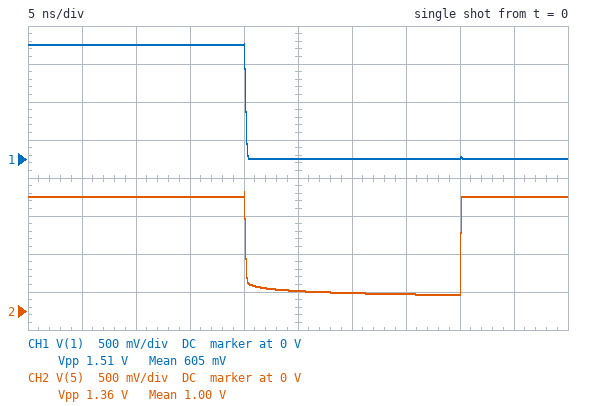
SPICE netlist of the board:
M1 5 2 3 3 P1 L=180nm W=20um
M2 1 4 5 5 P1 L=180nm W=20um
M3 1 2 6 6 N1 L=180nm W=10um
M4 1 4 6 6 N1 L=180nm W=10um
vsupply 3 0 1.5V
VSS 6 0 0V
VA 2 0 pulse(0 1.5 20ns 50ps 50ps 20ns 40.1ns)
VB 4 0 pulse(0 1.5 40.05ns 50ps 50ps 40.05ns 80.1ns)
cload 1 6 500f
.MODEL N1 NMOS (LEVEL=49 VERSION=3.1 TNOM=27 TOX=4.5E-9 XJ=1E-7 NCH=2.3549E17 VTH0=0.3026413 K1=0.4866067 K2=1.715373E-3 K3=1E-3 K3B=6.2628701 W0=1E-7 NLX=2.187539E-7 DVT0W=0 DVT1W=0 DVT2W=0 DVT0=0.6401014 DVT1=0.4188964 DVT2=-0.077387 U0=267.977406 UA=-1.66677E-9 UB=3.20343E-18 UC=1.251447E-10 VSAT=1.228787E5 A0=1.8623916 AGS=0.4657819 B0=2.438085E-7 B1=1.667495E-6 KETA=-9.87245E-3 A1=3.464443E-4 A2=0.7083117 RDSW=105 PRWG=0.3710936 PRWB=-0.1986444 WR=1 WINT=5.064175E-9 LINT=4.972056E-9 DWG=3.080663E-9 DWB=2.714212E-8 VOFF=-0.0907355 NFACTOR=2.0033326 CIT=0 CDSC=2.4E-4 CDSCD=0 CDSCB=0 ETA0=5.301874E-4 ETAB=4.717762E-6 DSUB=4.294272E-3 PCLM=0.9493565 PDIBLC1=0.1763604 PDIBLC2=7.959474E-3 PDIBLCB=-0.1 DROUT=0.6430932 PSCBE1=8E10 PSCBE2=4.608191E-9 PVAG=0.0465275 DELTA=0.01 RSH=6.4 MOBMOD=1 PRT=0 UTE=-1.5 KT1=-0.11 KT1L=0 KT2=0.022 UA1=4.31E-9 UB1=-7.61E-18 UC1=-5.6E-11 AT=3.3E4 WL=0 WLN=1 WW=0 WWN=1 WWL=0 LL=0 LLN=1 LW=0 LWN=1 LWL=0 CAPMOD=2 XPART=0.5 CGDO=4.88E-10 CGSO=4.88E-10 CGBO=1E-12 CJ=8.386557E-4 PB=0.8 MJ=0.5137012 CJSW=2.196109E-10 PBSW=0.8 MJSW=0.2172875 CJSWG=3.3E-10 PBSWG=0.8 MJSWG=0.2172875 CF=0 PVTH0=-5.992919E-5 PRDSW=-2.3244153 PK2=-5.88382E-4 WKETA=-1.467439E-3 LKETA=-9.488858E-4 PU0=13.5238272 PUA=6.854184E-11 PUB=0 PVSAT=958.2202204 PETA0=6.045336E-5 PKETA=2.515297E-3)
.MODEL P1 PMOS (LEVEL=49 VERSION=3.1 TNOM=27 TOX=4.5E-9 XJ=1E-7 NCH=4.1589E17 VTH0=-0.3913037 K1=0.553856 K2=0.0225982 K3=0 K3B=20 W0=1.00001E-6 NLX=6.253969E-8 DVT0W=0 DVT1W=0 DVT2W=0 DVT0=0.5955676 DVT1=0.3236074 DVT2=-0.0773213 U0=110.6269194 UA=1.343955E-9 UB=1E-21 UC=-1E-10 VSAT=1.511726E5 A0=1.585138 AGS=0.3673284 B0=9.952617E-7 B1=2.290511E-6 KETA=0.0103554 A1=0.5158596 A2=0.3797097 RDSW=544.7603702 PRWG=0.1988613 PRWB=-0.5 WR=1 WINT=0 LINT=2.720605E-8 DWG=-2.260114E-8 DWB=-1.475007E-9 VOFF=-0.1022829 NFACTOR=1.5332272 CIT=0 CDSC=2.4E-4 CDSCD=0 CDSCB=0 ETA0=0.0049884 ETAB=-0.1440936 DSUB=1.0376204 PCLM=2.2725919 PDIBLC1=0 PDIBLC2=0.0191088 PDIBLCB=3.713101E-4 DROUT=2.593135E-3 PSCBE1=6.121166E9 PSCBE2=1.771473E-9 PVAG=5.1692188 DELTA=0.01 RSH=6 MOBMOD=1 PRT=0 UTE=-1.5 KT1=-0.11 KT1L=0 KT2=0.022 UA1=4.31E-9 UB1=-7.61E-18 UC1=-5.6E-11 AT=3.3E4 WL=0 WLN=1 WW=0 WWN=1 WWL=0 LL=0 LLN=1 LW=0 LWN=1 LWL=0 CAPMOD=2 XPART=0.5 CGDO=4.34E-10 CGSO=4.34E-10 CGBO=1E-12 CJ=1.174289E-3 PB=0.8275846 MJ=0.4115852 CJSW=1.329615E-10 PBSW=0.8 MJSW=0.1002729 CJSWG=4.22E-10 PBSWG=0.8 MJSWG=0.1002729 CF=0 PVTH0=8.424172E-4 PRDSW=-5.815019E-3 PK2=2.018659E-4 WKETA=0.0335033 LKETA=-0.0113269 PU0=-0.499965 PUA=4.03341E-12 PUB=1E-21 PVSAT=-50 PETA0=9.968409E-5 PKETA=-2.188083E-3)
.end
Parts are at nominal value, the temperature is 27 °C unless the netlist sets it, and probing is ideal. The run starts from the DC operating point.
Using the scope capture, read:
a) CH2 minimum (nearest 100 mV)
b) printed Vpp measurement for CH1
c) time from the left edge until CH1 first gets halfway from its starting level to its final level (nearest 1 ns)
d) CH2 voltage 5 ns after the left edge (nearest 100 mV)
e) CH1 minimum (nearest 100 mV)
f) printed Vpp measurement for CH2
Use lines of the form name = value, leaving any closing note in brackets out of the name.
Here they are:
CH2 minimum = 200 mV
printed Vpp measurement for CH1 = 1.51 V
time from the left edge until CH1 first gets halfway from its starting level to its final level = 20 ns
CH2 voltage 5 ns after the left edge = 1.5 V
CH1 minimum = 0 V
printed Vpp measurement for CH2 = 1.36 V
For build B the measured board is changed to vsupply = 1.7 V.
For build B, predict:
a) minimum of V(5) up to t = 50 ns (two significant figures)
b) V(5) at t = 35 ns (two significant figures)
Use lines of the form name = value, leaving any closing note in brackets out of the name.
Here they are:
minimum of V(5) up to t = 50 ns = 230 mV
V(5) at t = 35 ns = 240 mV
